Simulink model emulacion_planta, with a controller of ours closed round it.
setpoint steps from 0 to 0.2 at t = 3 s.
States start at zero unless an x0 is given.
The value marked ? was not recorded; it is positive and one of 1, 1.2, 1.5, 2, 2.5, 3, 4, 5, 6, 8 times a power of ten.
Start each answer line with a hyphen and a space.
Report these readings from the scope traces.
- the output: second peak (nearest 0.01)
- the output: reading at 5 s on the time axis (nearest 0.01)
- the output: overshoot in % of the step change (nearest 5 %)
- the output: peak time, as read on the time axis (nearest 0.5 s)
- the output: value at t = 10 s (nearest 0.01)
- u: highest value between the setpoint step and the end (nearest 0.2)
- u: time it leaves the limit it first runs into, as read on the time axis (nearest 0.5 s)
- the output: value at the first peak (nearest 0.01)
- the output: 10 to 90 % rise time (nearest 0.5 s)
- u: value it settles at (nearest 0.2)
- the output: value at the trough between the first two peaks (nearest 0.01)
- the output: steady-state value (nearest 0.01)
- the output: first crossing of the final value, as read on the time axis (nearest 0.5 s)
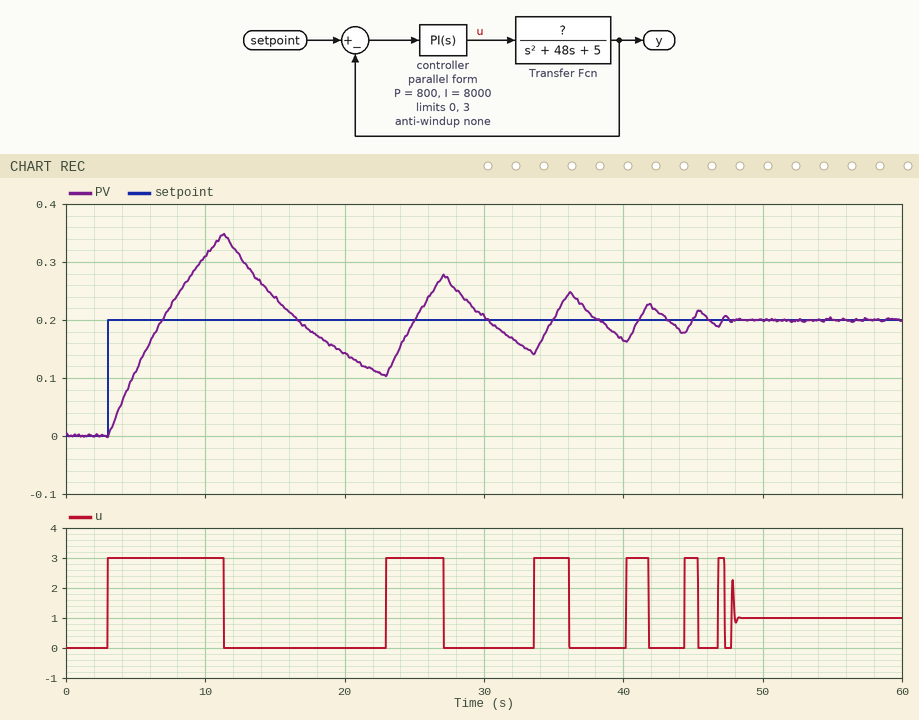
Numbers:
- 0.28
- 0.11
- 75 %
- 11.5 s
- 0.31
- 3.0
- 11.5 s
- 0.35
- 3.0 s
- 1.0
- 0.10
- 0.20
- 7.0 s
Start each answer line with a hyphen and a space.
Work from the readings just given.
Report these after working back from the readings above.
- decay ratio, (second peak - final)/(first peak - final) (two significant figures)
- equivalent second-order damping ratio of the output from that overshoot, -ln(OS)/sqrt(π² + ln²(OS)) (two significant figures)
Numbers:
- 0.53
- 0.091
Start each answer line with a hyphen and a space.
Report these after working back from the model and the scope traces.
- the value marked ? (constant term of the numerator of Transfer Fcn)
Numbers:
- 1
